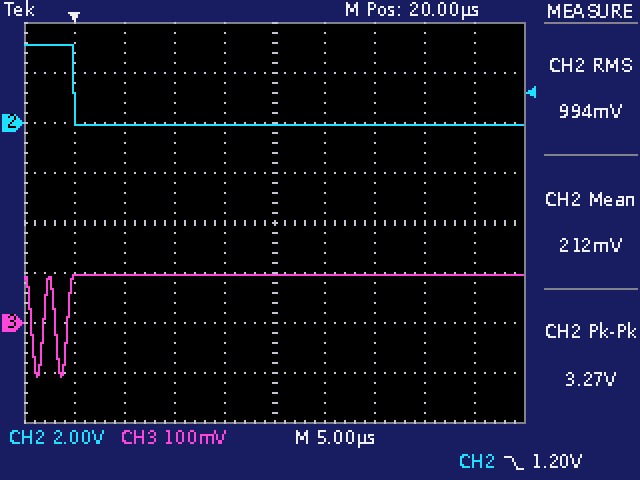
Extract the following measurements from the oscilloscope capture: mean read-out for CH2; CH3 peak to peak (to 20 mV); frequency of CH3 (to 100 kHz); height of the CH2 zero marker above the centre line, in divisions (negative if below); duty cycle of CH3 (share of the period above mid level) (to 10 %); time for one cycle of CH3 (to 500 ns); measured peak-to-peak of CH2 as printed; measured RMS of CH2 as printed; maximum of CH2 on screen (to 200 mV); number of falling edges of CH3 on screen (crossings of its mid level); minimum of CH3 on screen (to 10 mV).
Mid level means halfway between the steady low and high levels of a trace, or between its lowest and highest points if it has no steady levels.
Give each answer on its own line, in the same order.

212 mV
200 mV
400 kHz
+2.0 div
50 %
2.5 µs
3.27 V
994 mV
3.2 V
2
-110 mV
